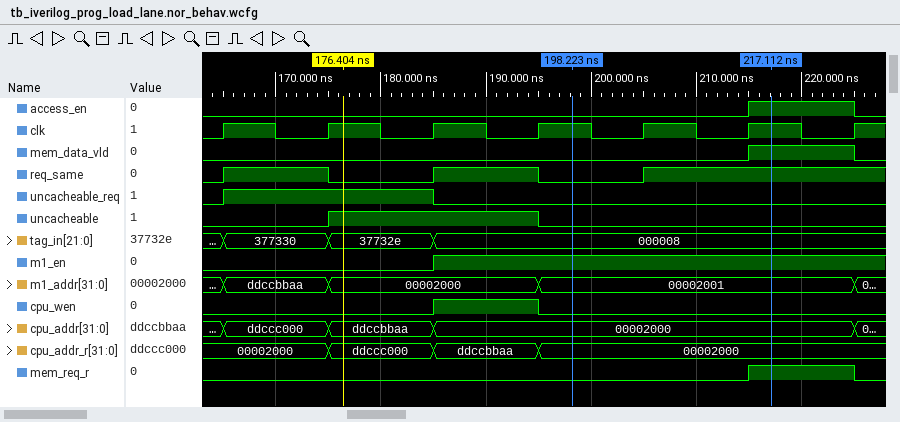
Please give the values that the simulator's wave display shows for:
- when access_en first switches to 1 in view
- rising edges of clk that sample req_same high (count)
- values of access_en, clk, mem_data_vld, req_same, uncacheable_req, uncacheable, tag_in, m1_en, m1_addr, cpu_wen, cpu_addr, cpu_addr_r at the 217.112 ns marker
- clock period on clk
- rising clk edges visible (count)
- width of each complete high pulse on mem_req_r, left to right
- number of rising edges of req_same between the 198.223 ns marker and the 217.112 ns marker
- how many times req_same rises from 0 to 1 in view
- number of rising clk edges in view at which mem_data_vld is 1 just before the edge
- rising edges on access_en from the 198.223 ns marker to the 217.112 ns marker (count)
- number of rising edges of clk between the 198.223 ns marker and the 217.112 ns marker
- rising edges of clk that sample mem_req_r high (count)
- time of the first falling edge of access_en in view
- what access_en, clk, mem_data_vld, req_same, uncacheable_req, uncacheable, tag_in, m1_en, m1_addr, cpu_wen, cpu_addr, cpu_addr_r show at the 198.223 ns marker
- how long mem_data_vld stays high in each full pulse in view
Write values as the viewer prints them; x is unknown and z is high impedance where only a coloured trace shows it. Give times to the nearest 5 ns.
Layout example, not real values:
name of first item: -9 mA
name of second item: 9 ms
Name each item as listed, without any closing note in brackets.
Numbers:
when access_en first switches to 1 in view: 215 ns
rising edges of clk that sample req_same high: 4
values of access_en, clk, mem_data_vld, req_same, uncacheable_req, uncacheable, tag_in, m1_en, m1_addr, cpu_wen, cpu_addr, cpu_addr_r at the 217.112 ns marker: access_en=1, clk=1, mem_data_vld=1, req_same=1, uncacheable_req=0, uncacheable=0, tag_in=000008, m1_en=1, m1_addr=00002001, cpu_wen=0, cpu_addr=00002000, cpu_addr_r=00002000
clock period on clk: 10 ns
rising clk edges visible: 7
width of each complete high pulse on mem_req_r, left to right: 10 ns
number of rising edges of req_same between the 198.223 ns marker and the 217.112 ns marker: 1
how many times req_same rises from 0 to 1 in view: 3
number of rising clk edges in view at which mem_data_vld is 1 just before the edge: 1
rising edges on access_en from the 198.223 ns marker to the 217.112 ns marker: 1
number of rising edges of clk between the 198.223 ns marker and the 217.112 ns marker: 2
rising edges of clk that sample mem_req_r high: 1
time of the first falling edge of access_en in view: 225 ns
what access_en, clk, mem_data_vld, req_same, uncacheable_req, uncacheable, tag_in, m1_en, m1_addr, cpu_wen, cpu_addr, cpu_addr_r show at the 198.223 ns marker: access_en=0, clk=1, mem_data_vld=0, req_same=0, uncacheable_req=0, uncacheable=0, tag_in=000008, m1_en=1, m1_addr=00002001, cpu_wen=0, cpu_addr=00002000, cpu_addr_r=00002000
how long mem_data_vld stays high in each full pulse in view: 10 ns
